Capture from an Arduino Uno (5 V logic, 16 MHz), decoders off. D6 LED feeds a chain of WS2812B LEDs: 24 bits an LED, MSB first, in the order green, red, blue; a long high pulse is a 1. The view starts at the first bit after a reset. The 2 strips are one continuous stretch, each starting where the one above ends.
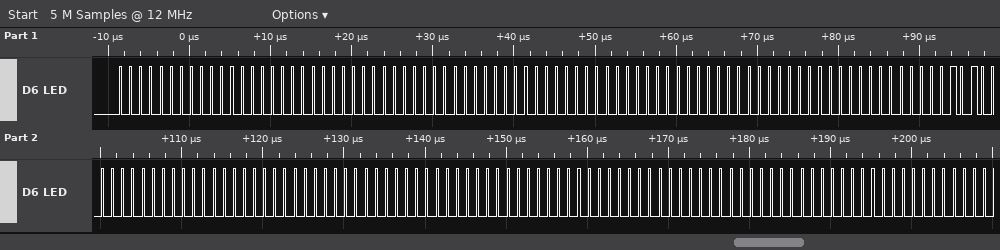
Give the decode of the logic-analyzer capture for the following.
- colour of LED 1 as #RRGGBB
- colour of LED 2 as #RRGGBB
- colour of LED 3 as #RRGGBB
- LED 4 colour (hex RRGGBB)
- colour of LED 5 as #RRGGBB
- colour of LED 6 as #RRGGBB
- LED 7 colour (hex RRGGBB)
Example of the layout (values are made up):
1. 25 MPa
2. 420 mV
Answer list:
1. #000000
2. #000000
3. #000000
4. #280000
5. #000000
6. #000000
7. #000000
